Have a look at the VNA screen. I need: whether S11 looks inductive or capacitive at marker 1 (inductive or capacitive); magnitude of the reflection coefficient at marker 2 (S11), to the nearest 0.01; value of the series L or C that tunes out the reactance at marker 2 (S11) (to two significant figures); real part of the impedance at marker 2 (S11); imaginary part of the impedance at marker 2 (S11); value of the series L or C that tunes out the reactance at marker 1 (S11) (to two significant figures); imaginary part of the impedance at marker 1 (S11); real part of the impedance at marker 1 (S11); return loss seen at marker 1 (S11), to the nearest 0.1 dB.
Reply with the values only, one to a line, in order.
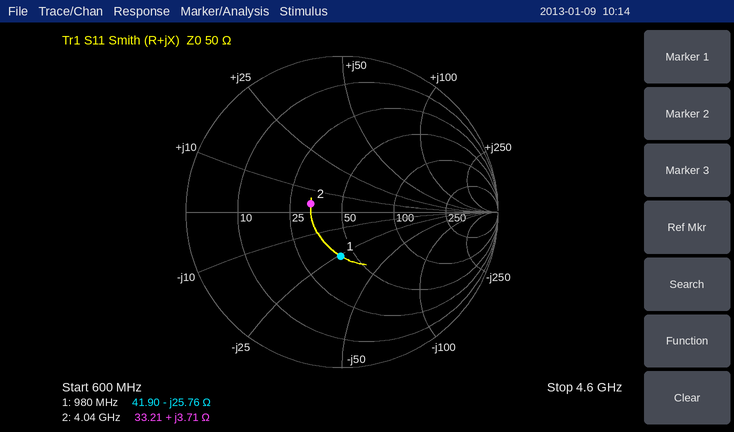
capacitive
0.21
11 pF
33.21 Ω
+3.71 Ω
4.2 nH
-25.76 Ω
41.90 Ω
11.0 dB
